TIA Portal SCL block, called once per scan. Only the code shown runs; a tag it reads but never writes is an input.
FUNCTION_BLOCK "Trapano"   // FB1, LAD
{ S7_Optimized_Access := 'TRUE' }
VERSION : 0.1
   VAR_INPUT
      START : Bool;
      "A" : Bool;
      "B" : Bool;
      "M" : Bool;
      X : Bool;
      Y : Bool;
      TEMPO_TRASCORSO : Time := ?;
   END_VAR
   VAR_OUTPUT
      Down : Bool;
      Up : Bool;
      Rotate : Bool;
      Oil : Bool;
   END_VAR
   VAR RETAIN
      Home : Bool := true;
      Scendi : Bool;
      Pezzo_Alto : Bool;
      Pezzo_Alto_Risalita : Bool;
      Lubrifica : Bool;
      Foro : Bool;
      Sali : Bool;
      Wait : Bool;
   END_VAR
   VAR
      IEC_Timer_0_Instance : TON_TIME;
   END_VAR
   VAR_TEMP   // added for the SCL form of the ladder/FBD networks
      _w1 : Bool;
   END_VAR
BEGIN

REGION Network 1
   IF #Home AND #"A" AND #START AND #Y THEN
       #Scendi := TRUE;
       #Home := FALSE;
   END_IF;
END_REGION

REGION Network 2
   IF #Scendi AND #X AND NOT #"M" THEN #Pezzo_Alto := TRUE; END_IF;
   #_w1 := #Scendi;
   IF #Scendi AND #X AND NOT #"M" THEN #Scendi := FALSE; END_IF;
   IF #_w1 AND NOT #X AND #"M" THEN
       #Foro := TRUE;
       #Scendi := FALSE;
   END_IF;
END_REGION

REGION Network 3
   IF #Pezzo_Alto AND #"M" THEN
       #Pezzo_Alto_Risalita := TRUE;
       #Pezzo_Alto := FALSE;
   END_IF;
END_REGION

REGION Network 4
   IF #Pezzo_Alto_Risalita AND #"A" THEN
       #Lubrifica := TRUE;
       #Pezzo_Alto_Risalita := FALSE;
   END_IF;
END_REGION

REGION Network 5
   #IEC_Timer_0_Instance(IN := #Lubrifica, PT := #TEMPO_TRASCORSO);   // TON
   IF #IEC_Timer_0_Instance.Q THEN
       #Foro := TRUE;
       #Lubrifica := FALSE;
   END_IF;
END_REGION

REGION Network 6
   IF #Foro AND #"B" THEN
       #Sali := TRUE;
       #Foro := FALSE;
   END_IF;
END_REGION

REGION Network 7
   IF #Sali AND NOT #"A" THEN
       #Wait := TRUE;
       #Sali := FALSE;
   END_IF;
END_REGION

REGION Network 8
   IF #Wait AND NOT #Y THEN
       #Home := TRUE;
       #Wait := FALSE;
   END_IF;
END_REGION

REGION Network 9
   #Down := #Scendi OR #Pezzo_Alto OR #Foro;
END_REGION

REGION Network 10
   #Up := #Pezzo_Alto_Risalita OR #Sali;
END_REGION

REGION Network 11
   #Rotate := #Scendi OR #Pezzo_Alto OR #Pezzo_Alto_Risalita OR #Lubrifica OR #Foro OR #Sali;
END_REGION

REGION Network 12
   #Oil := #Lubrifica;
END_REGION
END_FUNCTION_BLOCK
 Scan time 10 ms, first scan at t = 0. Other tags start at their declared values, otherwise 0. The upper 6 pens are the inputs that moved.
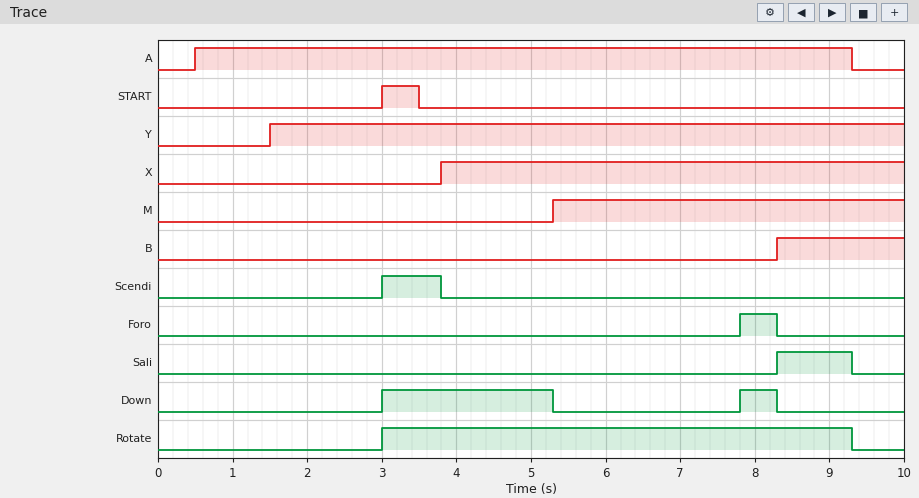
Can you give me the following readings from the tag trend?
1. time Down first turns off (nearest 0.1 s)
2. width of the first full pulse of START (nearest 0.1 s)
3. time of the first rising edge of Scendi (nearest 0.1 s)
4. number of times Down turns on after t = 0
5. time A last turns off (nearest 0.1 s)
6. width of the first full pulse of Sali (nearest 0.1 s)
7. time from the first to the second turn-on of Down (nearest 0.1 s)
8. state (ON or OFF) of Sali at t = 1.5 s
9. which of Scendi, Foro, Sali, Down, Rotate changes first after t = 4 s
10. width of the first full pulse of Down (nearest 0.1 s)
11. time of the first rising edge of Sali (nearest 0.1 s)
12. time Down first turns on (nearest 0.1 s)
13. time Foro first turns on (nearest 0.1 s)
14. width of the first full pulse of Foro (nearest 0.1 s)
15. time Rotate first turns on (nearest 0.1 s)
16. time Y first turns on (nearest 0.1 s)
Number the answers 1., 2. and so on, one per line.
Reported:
1. 5.3 s
2. 0.5 s
3. 3.0 s
4. 2
5. 9.3 s
6. 1.0 s
7. 4.8 s
8. OFF
9. Down
10. 2.3 s
11. 8.3 s
12. 3.0 s
13. 7.8 s
14. 0.5 s
15. 3.0 s
16. 1.5 s
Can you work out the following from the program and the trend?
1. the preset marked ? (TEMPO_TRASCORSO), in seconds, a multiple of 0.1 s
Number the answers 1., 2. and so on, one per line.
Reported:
1. 2.5 s
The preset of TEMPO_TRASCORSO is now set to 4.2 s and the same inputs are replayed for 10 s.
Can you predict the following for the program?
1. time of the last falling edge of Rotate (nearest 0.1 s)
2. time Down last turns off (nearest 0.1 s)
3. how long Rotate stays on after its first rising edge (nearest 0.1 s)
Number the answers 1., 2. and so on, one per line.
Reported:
1. 9.5 s
2. 5.3 s
3. 6.5 s
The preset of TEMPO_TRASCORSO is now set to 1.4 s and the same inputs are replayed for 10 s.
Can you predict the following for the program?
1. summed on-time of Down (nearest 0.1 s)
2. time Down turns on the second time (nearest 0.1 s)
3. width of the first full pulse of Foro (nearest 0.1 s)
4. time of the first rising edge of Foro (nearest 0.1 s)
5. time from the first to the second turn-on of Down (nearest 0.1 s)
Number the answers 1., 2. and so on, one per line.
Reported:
1. 3.9 s
2. 6.7 s
3. 1.6 s
4. 6.7 s
5. 3.7 s
